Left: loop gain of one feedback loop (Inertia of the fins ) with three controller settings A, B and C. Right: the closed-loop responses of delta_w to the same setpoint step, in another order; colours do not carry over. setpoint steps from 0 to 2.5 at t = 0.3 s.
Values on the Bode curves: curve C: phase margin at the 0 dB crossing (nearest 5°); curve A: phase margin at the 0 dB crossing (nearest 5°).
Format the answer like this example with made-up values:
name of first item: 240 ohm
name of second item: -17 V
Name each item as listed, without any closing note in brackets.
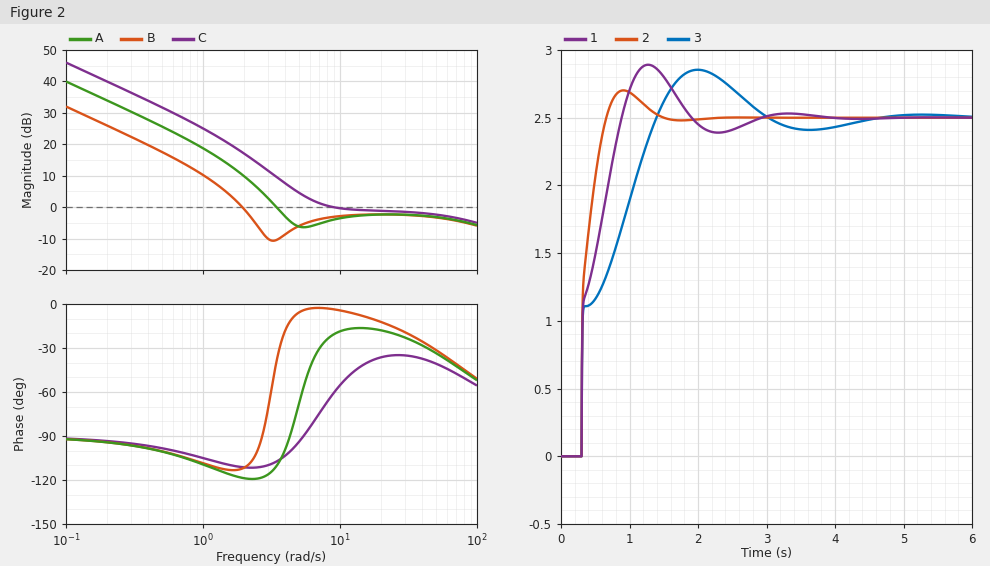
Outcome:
curve C: phase margin at the 0 dB crossing: 120°
curve A: phase margin at the 0 dB crossing: 70°
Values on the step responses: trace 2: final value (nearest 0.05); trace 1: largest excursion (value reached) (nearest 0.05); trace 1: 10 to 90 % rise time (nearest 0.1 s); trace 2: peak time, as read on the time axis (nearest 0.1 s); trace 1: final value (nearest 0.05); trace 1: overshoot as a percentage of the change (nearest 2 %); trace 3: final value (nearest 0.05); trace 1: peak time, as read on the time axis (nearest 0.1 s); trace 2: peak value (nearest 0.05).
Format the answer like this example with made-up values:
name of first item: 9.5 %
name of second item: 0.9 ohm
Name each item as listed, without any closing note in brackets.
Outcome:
trace 2: final value: 2.50
trace 1: largest excursion (value reached): 2.90
trace 1: 10 to 90 % rise time: 0.5 s
trace 2: peak time, as read on the time axis: 0.9 s
trace 1: final value: 2.50
trace 1: overshoot as a percentage of the change: 16 %
trace 3: final value: 2.50
trace 1: peak time, as read on the time axis: 1.3 s
trace 2: peak value: 2.70
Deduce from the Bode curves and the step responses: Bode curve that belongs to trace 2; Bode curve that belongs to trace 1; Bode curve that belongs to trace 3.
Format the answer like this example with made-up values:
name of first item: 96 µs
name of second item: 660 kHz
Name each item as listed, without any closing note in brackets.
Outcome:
Bode curve that belongs to trace 2: C
Bode curve that belongs to trace 1: A
Bode curve that belongs to trace 3: B
